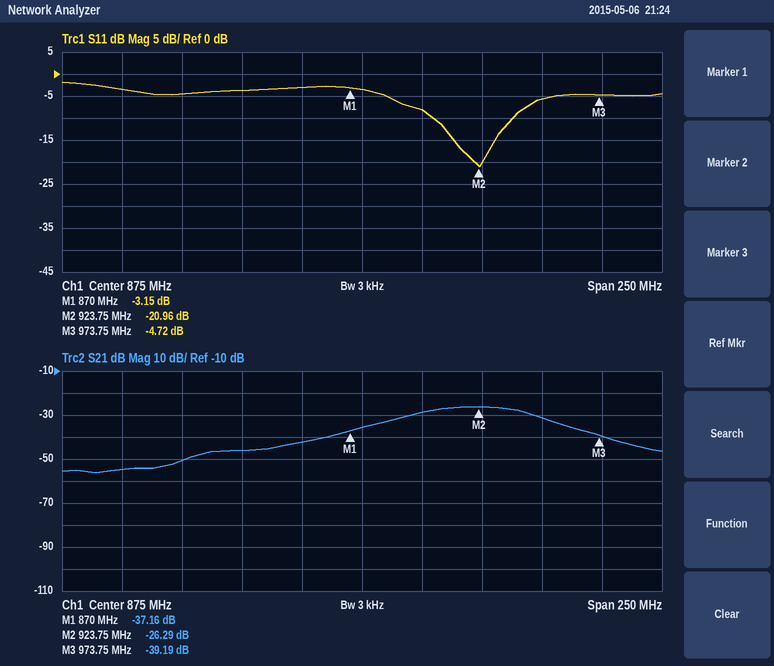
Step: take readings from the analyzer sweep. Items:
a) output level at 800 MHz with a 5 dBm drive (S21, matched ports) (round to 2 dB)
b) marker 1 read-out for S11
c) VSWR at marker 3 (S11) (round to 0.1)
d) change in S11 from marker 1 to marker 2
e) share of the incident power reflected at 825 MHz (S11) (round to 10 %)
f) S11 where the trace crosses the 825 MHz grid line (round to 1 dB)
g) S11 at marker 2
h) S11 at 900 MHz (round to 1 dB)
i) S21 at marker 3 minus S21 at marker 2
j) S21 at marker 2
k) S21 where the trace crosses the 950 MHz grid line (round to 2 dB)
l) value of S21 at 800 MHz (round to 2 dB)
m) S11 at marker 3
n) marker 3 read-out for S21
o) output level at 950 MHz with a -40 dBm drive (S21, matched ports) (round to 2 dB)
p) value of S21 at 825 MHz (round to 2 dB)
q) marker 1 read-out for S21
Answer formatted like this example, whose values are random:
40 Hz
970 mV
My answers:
-46 dBm
-3.15 dB
3.8
-17.81 dB
40 %
-4 dB
-20.96 dB
-8 dB
-12.90 dB
-26.29 dB
-32 dB
-50 dB
-4.72 dB
-39.19 dB
-72 dBm
-46 dB
-37.16 dB
